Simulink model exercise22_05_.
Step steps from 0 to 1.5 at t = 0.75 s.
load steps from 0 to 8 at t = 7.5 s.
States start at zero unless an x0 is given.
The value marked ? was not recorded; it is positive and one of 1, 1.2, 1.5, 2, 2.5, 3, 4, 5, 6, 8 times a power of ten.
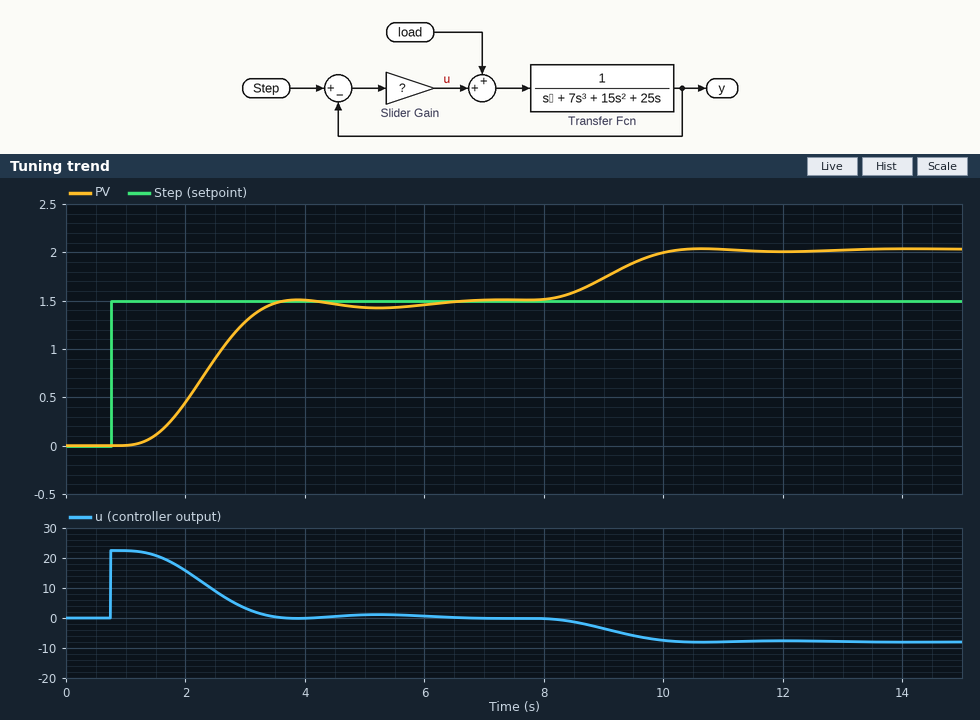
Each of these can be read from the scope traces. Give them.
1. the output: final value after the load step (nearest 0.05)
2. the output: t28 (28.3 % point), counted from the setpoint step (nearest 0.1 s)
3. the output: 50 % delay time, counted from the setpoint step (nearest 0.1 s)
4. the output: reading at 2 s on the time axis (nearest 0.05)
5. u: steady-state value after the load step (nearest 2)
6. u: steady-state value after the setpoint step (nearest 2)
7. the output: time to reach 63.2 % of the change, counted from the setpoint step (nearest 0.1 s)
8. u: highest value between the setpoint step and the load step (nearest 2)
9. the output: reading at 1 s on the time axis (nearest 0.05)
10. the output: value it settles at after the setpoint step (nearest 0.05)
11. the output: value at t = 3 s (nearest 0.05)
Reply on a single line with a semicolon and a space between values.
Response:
2.05; 1.2 s; 1.6 s; 0.45; -8; 0; 1.8 s; 22; 0.00; 1.50; 1.30
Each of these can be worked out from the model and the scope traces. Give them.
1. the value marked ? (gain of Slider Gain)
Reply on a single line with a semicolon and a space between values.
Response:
15
